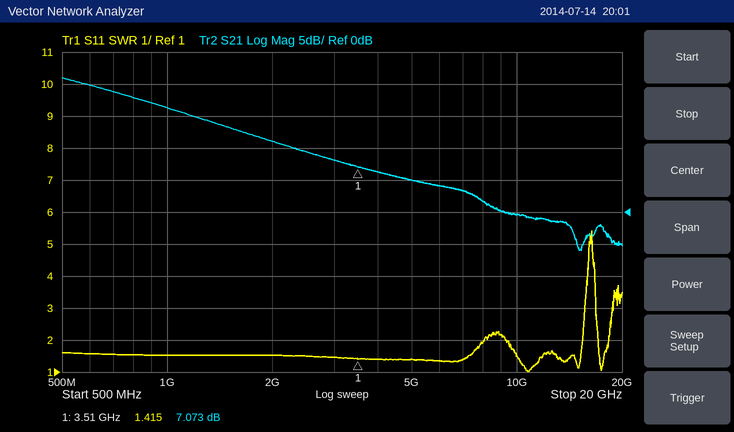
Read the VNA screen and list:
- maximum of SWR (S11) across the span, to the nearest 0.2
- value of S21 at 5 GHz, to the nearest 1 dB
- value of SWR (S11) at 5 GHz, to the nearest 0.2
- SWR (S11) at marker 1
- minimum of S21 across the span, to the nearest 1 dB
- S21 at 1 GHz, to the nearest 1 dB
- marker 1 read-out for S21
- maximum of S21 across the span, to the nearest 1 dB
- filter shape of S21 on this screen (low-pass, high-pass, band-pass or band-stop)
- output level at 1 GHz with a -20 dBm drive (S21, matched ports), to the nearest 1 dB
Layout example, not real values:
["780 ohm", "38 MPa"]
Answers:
["5.4", "5 dB", "1.4", "1.415", "-6 dB", "16 dB", "7.073 dB", "21 dB", "low-pass", "-4 dBm"]
